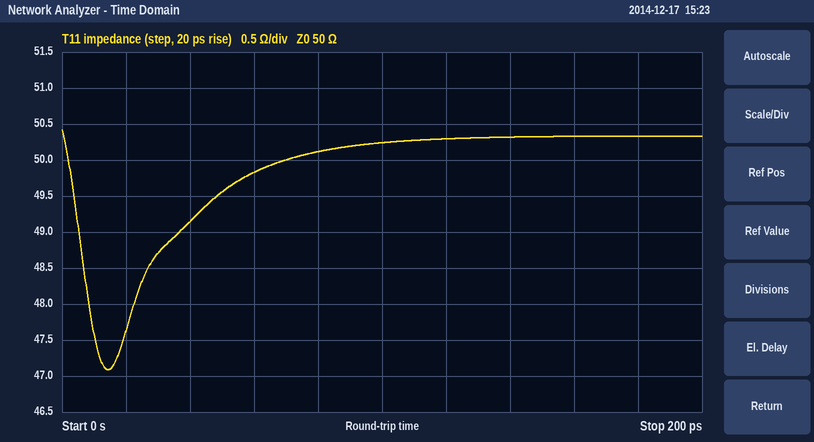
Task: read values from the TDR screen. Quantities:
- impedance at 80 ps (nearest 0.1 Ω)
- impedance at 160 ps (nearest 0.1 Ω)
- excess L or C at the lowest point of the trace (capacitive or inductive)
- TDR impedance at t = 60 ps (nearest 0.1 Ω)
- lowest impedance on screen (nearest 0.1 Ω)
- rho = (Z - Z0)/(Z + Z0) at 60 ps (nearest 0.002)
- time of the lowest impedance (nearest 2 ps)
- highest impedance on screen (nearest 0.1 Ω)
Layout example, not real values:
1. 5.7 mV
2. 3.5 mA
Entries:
1. 50.1 Ω
2. 50.3 Ω
3. capacitive
4. 49.8 Ω
5. 47.1 Ω
6. -0.002
7. 14 ps
8. 50.4 Ω
